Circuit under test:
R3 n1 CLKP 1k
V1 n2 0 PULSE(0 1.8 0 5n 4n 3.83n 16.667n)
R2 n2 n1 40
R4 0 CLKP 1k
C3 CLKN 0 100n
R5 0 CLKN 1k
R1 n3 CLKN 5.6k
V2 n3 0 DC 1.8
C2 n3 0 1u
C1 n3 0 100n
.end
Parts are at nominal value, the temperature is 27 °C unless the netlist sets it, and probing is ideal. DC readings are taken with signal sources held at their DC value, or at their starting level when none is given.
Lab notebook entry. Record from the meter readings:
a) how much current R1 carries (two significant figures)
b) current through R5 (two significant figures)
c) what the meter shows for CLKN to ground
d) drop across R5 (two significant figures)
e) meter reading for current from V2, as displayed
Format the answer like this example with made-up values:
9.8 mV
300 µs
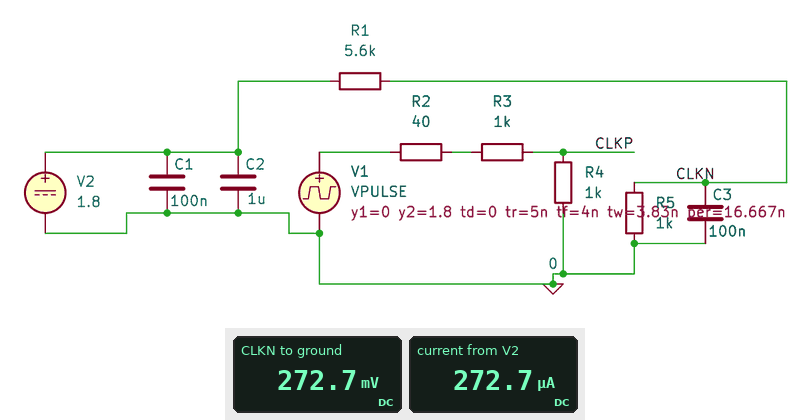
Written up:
270 µA
270 µA
272.7 mV
270 mV
272.7 µA
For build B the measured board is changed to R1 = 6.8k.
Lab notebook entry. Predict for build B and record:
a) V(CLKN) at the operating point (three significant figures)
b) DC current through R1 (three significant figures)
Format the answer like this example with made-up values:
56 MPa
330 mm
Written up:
231 mV
231 µA
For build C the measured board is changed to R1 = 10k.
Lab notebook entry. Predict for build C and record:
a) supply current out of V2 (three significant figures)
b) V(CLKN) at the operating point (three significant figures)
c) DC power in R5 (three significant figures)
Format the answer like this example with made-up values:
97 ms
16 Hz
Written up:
164 µA
164 mV
26.8 µW
